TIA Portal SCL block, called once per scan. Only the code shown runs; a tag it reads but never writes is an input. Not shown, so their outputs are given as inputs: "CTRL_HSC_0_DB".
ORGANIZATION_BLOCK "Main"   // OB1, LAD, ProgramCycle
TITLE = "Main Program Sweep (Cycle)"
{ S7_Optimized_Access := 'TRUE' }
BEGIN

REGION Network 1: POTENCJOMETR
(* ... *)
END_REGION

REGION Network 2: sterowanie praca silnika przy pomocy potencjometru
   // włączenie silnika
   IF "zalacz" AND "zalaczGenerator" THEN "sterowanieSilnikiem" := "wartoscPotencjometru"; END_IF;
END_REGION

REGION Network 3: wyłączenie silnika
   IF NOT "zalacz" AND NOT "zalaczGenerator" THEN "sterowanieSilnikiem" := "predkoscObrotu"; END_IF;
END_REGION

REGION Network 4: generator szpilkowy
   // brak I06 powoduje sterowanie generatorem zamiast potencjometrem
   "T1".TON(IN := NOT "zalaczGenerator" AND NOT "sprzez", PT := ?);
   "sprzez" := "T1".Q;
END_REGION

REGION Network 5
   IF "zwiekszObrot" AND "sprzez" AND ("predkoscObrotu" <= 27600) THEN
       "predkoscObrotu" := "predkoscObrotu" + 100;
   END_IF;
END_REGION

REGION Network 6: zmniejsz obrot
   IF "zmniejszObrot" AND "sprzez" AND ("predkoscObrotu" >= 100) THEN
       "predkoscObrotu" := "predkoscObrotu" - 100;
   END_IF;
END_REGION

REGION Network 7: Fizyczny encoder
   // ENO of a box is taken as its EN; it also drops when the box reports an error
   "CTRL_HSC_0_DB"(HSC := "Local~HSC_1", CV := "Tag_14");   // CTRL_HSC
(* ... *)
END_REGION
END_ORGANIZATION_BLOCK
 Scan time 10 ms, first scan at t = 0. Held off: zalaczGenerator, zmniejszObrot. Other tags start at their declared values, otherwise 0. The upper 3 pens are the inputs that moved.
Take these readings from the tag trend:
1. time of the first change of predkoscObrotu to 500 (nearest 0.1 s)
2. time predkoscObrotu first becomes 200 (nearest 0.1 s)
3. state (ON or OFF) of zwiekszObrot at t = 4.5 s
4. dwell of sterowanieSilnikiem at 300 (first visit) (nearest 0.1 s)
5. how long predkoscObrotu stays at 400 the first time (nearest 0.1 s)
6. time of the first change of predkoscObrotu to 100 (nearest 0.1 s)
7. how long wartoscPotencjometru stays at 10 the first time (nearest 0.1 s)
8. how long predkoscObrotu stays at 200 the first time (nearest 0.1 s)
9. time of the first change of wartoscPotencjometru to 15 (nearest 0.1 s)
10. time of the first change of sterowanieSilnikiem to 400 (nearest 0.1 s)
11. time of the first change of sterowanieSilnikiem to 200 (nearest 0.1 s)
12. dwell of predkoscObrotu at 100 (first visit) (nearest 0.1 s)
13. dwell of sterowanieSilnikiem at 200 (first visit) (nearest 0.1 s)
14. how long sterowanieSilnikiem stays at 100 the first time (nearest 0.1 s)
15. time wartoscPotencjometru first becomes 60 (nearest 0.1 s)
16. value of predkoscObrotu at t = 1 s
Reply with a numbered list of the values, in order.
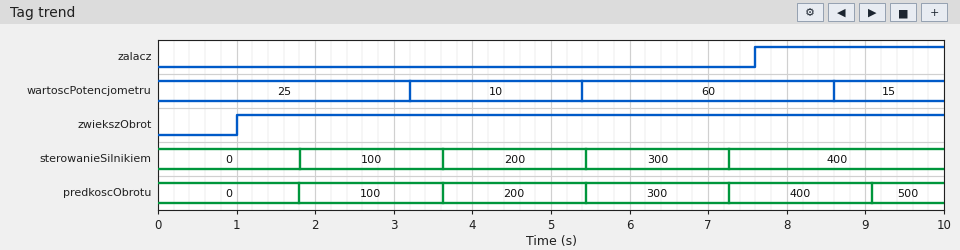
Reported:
1. 9.1 s
2. 3.6 s
3. ON
4. 1.8 s
5. 1.8 s
6. 1.8 s
7. 2.2 s
8. 1.8 s
9. 8.6 s
10. 7.3 s
11. 3.6 s
12. 1.8 s
13. 1.8 s
14. 1.8 s
15. 5.4 s
16. 0
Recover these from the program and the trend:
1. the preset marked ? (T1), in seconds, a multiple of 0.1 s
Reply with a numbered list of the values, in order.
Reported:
1. 1.8 s
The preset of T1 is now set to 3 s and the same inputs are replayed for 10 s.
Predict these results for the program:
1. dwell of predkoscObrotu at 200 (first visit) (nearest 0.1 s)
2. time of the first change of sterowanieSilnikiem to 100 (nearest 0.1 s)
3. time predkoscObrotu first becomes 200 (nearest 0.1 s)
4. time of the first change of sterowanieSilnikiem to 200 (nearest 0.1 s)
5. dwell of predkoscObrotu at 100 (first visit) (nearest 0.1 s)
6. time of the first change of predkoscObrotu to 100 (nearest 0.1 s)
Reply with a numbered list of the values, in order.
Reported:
1. 3.0 s
2. 3.0 s
3. 6.0 s
4. 6.0 s
5. 3.0 s
6. 3.0 s
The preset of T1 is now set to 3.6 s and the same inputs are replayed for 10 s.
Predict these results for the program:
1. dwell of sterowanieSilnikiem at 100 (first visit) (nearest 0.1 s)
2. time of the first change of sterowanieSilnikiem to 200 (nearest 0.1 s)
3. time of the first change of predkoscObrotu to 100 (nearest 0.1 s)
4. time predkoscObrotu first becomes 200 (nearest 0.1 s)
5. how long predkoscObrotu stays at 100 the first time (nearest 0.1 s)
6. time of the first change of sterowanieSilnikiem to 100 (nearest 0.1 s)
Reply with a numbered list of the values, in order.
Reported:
1. 3.6 s
2. 7.2 s
3. 3.6 s
4. 7.2 s
5. 3.6 s
6. 3.6 s
